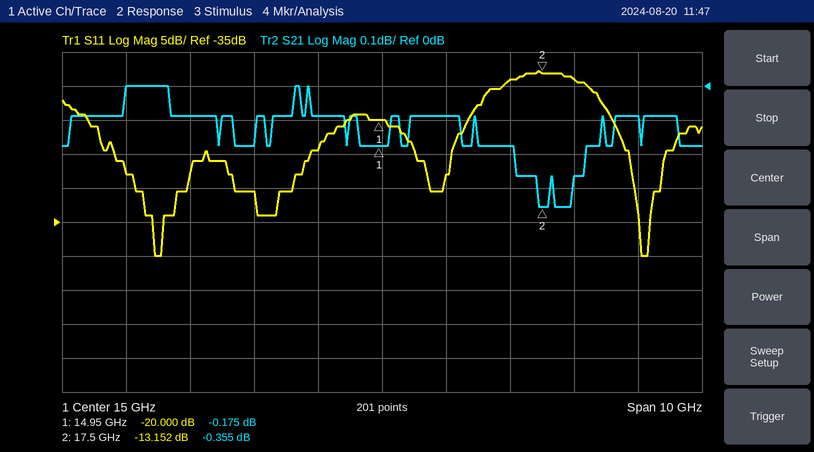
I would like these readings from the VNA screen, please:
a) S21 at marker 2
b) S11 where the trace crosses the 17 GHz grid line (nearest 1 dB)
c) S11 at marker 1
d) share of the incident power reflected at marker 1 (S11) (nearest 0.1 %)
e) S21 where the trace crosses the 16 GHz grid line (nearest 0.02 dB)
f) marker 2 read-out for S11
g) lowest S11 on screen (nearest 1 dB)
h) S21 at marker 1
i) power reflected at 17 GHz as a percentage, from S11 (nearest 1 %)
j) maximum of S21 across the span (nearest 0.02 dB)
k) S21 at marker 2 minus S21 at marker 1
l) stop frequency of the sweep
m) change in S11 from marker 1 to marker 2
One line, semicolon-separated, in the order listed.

-0.355 dB; -14 dB; -20.000 dB; 1.0 %; -0.08 dB; -13.152 dB; -40 dB; -0.175 dB; 4 %; 0.00 dB; -0.180 dB; 20 GHz; 6.848 dB
